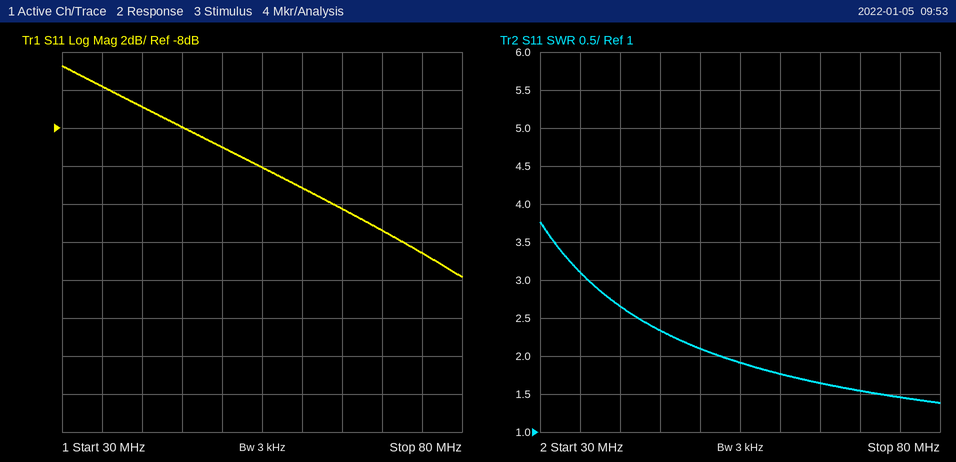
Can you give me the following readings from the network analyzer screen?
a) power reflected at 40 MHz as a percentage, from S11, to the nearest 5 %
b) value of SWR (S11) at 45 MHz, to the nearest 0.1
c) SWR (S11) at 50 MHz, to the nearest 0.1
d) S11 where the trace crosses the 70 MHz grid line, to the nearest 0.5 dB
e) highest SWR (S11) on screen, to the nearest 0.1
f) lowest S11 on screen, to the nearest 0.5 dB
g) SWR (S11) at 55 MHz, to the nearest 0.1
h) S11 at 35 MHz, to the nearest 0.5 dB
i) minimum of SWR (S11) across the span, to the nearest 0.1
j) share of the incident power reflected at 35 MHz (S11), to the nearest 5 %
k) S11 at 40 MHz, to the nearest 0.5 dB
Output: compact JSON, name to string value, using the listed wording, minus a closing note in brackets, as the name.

{"power reflected at 40 MHz as a percentage, from S11, to the nearest 5 %": "20 %", "value of SWR (S11) at 45 MHz, to the nearest 0.1": "2.3", "SWR (S11) at 50 MHz, to the nearest 0.1": "2.1", "S11 where the trace crosses the 70 MHz grid line, to the nearest 0.5 dB": "-13.5 dB", "highest SWR (S11) on screen, to the nearest 0.1": "3.8", "lowest S11 on screen, to the nearest 0.5 dB": "-16.0 dB", "SWR (S11) at 55 MHz, to the nearest 0.1": "1.9", "S11 at 35 MHz, to the nearest 0.5 dB": "-6.0 dB", "minimum of SWR (S11) across the span, to the nearest 0.1": "1.4", "share of the incident power reflected at 35 MHz (S11), to the nearest 5 %": "25 %", "S11 at 40 MHz, to the nearest 0.5 dB": "-7.0 dB"}
